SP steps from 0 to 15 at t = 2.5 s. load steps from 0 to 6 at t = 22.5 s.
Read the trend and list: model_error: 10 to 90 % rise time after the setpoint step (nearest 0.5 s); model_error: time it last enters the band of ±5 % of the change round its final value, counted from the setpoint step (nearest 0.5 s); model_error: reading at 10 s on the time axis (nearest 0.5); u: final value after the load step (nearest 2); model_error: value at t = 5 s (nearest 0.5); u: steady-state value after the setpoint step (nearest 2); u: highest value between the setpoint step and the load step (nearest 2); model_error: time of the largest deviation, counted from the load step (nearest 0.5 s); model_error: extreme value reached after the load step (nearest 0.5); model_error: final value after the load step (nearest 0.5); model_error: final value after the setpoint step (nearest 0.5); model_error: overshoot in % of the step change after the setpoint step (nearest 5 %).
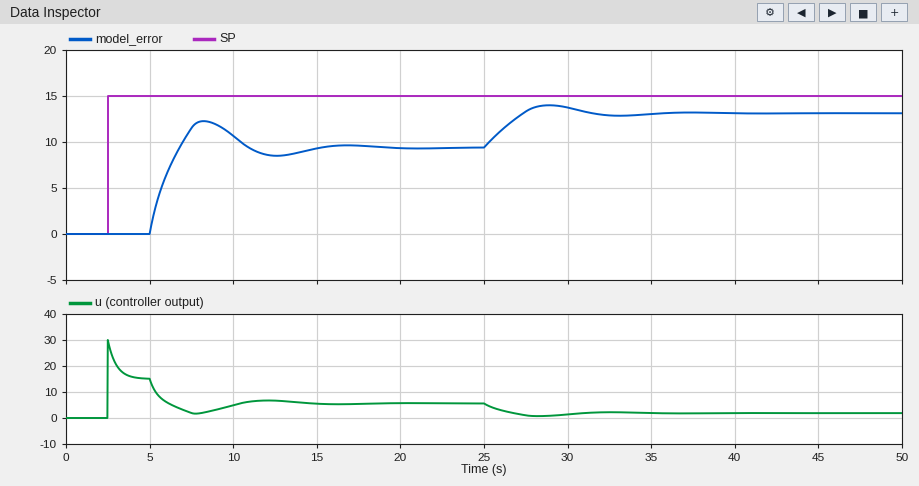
1.5 s
11.5 s
10.5
2
0.0
6
30
6.5 s
14.0
13.0
9.5
30 %
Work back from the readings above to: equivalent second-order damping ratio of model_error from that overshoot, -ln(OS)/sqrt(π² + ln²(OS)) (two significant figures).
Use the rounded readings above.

0.36
